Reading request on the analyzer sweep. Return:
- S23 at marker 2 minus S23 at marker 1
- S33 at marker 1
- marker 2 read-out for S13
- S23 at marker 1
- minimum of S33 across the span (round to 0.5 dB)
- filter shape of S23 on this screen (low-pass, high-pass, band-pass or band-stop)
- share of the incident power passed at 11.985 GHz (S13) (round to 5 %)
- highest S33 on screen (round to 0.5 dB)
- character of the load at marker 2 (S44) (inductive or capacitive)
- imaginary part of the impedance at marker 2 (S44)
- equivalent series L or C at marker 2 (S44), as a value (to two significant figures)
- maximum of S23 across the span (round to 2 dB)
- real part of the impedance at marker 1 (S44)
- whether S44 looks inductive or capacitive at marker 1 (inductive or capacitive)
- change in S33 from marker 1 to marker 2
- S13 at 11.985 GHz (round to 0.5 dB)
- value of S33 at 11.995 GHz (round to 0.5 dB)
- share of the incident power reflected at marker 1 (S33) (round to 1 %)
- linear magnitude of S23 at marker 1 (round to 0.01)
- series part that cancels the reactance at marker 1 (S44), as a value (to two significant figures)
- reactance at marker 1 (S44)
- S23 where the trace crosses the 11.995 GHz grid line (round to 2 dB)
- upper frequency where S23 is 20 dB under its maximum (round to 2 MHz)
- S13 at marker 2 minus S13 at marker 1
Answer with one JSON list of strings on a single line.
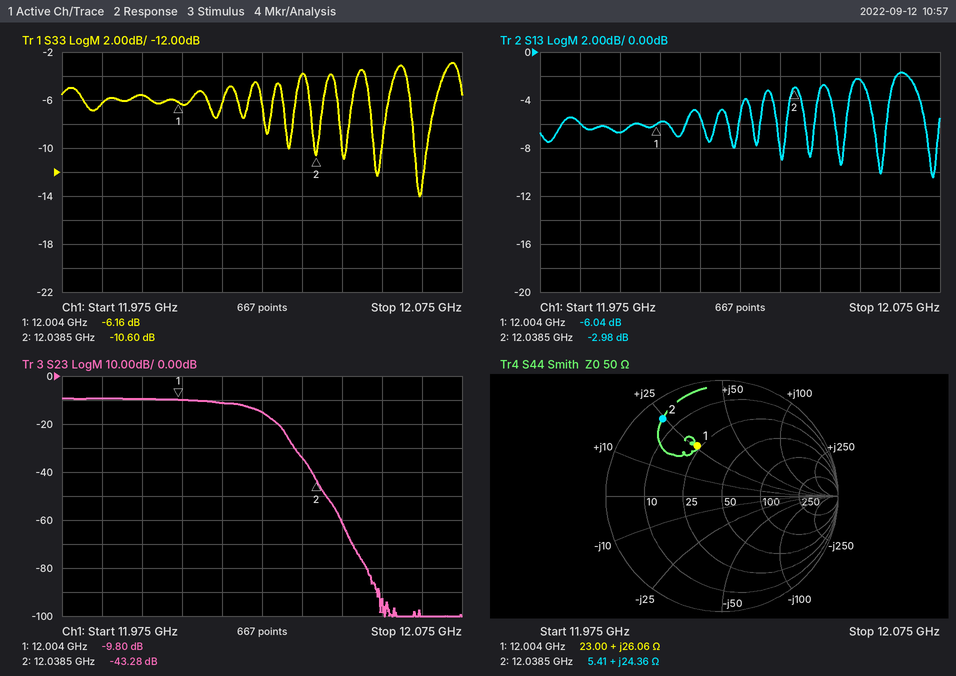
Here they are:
["-33.48 dB", "-6.16 dB", "-2.98 dB", "-9.80 dB", "-14.0 dB", "low-pass", "25 %", "-3.0 dB", "inductive", "+24.36 Ω", "320 pH", "-10 dB", "23.00 Ω", "inductive", "-4.44 dB", "-6.0 dB", "-5.5 dB", "24 %", "0.32", "510 fF", "+26.06 Ω", "-10 dB", "12.032 GHz", "3.06 dB"]
